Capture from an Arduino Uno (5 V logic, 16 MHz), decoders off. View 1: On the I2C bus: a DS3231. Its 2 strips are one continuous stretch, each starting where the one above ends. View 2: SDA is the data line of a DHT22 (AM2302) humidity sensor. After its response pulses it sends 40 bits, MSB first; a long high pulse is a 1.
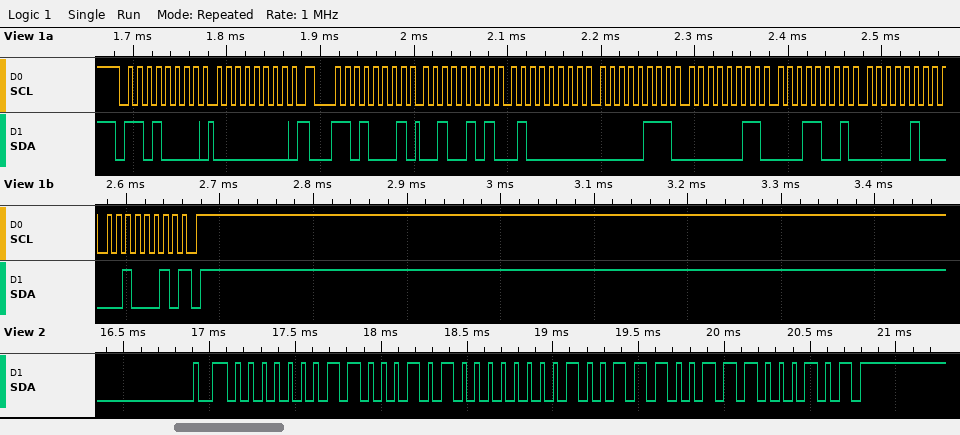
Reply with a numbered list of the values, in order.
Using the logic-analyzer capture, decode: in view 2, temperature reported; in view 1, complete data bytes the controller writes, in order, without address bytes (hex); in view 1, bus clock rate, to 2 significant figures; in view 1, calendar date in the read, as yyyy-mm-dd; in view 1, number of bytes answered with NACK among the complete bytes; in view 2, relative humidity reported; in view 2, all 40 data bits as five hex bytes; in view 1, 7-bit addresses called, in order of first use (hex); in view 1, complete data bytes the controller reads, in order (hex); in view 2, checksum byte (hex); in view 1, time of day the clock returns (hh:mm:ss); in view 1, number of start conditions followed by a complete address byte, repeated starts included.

1. 31.3 °C
2. 00
3. 100 kHz
4. 2022-04-19
5. 1
6. 39.4 %
7. 01 8A 01 39 C5
8. 0x68
9. 25 40 07 03 19 04 22
10. 0xC5
11. 07:40:25
12. 2
